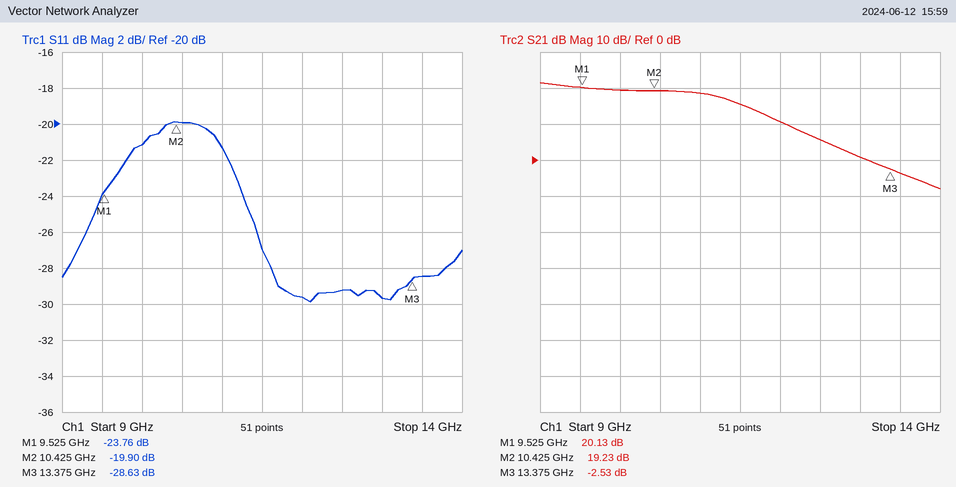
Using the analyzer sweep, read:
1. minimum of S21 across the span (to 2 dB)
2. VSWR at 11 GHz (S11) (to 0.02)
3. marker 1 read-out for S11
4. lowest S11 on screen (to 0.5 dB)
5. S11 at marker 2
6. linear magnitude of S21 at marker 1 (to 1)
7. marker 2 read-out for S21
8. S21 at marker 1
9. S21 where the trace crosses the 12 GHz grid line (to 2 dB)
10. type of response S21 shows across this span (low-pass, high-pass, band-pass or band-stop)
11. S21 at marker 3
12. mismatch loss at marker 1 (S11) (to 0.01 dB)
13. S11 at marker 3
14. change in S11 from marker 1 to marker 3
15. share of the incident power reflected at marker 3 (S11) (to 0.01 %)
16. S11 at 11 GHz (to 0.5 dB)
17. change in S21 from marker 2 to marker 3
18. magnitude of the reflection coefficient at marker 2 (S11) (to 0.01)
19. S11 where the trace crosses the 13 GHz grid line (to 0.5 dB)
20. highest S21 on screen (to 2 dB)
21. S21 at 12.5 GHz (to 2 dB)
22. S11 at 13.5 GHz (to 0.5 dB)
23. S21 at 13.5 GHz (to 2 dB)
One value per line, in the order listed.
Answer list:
-8 dB
1.18
-23.76 dB
-30.0 dB
-19.90 dB
10
19.23 dB
20.13 dB
10 dB
low-pass
-2.53 dB
0.02 dB
-28.63 dB
-4.87 dB
0.14 %
-21.5 dB
-21.76 dB
0.10
-29.5 dB
22 dB
6 dB
-28.5 dB
-4 dB
